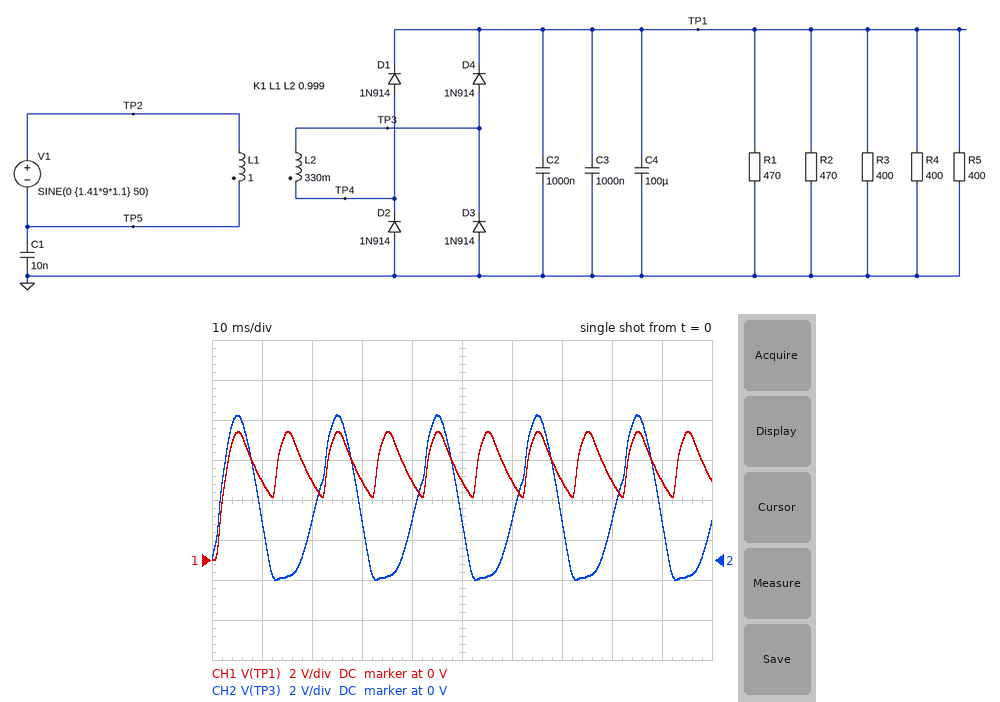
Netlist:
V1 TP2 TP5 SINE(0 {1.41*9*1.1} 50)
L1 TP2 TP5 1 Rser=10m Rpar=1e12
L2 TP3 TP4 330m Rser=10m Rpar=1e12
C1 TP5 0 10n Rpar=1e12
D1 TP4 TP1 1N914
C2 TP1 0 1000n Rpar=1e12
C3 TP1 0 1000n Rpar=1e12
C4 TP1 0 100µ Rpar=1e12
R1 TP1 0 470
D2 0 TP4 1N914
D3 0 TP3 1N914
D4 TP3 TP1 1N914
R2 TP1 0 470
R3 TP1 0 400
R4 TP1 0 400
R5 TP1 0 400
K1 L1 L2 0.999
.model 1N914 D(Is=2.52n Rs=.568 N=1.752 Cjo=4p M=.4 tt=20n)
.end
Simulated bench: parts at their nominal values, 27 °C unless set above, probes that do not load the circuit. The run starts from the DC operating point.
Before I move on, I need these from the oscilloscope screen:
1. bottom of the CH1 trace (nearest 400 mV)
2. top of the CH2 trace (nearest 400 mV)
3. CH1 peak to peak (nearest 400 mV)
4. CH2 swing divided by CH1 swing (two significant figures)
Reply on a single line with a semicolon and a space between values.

0 V; 7.2 V; 6.4 V; 1.3
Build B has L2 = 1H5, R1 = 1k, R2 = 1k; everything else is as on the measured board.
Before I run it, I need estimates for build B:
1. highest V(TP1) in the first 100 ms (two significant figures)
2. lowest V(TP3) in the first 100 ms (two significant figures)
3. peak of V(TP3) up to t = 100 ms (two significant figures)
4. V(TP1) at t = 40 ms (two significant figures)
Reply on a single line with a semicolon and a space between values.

17 V; -1.3 V; 18 V; 11 V
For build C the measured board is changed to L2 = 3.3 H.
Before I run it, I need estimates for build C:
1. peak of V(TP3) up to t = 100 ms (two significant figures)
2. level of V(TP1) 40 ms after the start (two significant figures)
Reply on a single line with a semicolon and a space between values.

29 V; 18 V
